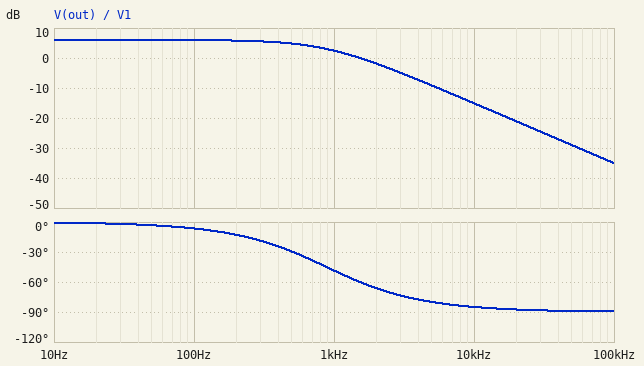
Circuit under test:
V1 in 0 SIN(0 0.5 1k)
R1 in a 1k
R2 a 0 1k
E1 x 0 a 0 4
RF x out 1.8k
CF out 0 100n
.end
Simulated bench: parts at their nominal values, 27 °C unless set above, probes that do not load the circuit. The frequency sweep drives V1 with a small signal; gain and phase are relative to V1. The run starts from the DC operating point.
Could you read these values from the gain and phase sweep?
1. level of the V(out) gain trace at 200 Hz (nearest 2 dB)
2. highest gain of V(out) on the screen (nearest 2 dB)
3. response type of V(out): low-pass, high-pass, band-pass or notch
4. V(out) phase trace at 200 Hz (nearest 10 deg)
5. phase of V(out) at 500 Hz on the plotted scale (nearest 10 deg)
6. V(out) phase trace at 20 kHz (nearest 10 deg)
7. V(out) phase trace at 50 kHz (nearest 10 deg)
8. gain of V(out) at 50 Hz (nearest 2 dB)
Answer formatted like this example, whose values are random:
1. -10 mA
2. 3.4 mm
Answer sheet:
1. 6 dB
2. 6 dB
3. low-pass
4. -10 deg
5. -30 deg
6. -90 deg
7. -90 deg
8. 6 dB
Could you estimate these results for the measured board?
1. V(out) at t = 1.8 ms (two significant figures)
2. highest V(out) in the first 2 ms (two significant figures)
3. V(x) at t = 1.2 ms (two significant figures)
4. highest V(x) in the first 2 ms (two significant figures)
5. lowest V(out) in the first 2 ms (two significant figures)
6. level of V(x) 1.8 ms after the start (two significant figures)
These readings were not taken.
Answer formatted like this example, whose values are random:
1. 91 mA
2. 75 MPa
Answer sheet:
1. -570 mV
2. 720 mV
3. 950 mV
4. 1.0 V
5. -660 mV
6. -950 mV
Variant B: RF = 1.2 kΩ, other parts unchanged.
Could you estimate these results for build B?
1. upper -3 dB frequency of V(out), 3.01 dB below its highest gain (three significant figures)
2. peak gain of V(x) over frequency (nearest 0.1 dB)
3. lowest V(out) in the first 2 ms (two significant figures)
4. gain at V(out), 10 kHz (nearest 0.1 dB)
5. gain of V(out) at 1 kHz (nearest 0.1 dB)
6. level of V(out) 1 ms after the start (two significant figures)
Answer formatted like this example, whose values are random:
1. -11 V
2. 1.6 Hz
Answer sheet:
1. 1.33 kHz
2. 6.0 dB
3. -800 mV
4. -11.6 dB
5. 4.1 dB
6. -480 mV
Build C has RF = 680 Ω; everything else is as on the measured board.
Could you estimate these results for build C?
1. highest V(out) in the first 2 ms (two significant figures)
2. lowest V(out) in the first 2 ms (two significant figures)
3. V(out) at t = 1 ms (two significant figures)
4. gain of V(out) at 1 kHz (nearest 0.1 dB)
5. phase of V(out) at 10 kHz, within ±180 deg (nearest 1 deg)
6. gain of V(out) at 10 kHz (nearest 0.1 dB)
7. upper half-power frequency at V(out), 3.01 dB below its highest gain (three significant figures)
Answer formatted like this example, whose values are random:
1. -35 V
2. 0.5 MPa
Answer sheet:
1. 920 mV
2. -920 mV
3. -360 mV
4. 5.3 dB
5. -77 deg
6. -6.8 dB
7. 2.34 kHz
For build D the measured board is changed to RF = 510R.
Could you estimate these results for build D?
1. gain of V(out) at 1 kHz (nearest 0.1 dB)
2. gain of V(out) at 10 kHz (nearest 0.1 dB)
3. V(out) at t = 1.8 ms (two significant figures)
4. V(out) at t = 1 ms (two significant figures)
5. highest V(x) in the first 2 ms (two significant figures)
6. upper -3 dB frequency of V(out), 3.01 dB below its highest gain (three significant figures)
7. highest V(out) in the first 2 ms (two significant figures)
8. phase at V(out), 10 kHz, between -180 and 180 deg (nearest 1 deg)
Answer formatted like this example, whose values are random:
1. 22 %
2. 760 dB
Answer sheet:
1. 5.6 dB
2. -4.5 dB
3. -950 mV
4. -290 mV
5. 1.0 V
6. 3.12 kHz
7. 950 mV
8. -73 deg
